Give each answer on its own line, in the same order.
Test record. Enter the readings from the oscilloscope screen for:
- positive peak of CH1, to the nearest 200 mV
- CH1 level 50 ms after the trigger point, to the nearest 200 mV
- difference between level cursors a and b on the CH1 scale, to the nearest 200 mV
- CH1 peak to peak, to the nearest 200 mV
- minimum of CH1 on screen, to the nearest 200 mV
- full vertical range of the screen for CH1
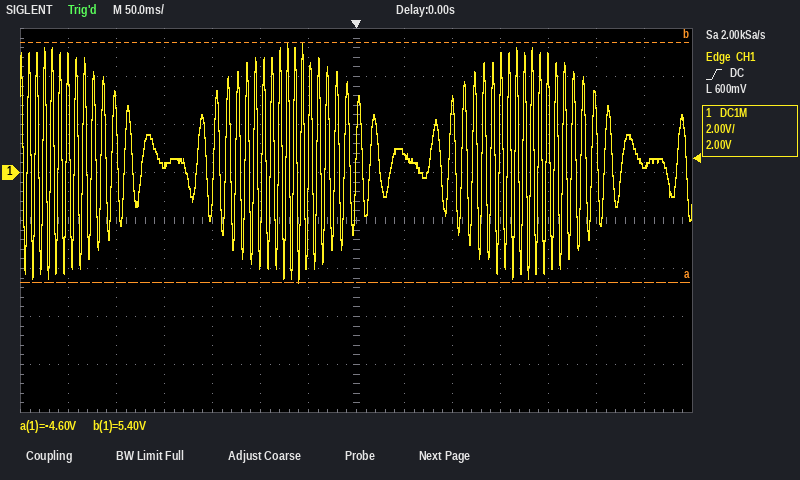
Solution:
5.4 V
800 mV
10.0 V
10.0 V
-4.6 V
16 V
